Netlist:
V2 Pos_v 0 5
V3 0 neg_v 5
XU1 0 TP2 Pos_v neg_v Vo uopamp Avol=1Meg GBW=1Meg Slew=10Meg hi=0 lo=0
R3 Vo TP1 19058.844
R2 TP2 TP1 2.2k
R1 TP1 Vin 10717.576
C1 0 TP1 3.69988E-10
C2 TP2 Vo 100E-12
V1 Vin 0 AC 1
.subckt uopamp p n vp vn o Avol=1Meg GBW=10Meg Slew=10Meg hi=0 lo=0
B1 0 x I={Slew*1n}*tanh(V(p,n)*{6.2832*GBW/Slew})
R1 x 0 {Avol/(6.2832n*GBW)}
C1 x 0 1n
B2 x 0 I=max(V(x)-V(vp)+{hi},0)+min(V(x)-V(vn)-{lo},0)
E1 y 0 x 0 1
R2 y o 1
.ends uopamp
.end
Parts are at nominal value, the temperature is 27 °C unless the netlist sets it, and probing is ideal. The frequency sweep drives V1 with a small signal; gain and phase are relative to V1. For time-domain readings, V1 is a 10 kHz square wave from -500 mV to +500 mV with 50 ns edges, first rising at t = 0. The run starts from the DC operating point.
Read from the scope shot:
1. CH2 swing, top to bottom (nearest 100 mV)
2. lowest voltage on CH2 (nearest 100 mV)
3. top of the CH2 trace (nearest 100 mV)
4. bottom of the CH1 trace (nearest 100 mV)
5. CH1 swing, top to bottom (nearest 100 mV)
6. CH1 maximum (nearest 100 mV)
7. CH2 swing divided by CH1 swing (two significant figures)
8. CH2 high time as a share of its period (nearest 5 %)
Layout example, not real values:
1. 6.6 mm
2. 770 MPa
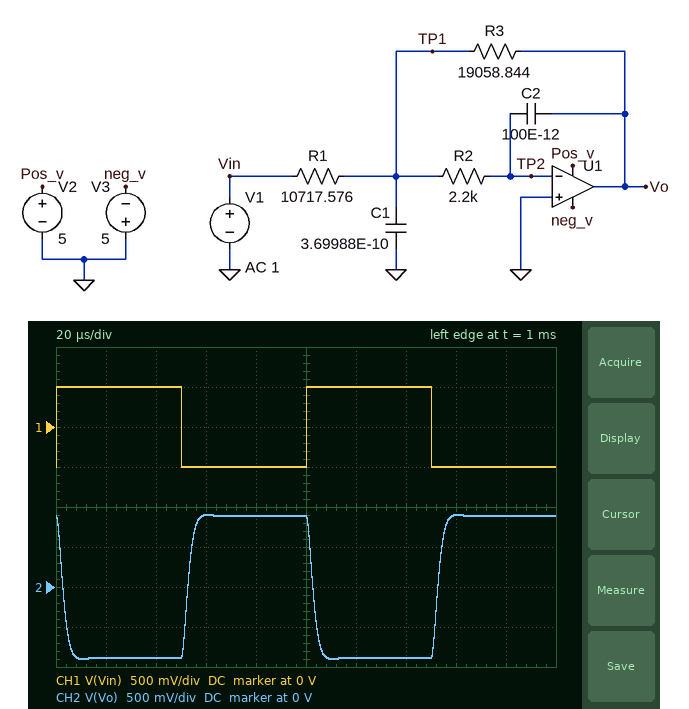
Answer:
1. 1.8 V
2. -900 mV
3. 900 mV
4. -500 mV
5. 1.0 V
6. 500 mV
7. 1.8
8. 50 %
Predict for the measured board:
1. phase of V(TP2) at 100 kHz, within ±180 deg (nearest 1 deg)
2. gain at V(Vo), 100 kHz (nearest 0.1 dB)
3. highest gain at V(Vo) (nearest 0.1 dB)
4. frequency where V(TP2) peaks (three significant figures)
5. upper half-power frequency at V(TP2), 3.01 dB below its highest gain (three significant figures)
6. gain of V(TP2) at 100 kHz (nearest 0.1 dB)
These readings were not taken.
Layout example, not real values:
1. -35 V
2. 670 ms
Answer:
1. -7 deg
2. -0.2 dB
3. 5.0 dB
4. 94.5 kHz
5. 204 kHz
6. -20.2 dB
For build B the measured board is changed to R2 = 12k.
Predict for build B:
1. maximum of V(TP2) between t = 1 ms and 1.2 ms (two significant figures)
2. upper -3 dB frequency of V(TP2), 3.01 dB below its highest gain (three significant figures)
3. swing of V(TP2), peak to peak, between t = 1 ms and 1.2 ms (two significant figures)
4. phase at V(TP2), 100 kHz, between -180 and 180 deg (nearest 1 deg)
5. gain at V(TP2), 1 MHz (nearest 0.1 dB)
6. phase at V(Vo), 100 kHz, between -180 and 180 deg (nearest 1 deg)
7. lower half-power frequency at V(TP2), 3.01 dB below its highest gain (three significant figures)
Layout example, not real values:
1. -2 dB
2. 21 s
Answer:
1. 36 mV
2. 114 kHz
3. 72 mV
4. -44 deg
5. -49.1 dB
6. 46 deg
7. 22.9 kHz
